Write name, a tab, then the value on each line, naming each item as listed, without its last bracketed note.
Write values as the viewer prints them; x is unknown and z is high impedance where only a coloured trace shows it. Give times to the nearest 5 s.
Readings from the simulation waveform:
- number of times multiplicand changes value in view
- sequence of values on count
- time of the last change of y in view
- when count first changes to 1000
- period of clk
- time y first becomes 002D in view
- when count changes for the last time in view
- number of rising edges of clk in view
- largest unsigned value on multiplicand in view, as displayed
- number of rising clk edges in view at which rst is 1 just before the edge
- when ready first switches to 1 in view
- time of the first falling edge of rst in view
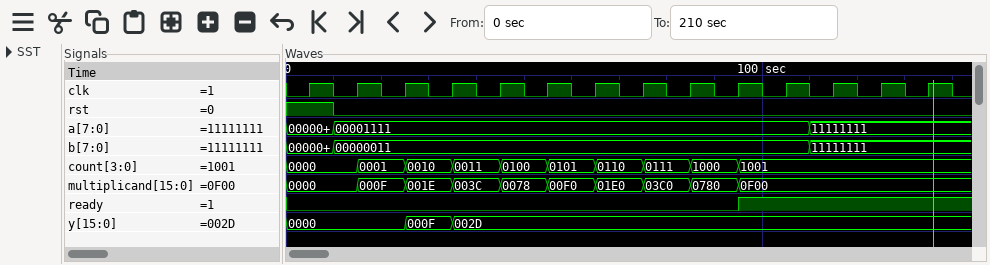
number of times multiplicand changes value in view	9
sequence of values on count	0000, 0001, 0010, 0011, 0100, 0101, 0110, 0111, 1000, 1001
time of the last change of y in view	35 s
when count first changes to 1000	85 s
period of clk	10 s
time y first becomes 002D in view	35 s
when count changes for the last time in view	95 s
number of rising edges of clk in view	14
largest unsigned value on multiplicand in view, as displayed	0F00
number of rising clk edges in view at which rst is 1 just before the edge	1
when ready first switches to 1 in view	95 s
time of the first falling edge of rst in view	10 s
